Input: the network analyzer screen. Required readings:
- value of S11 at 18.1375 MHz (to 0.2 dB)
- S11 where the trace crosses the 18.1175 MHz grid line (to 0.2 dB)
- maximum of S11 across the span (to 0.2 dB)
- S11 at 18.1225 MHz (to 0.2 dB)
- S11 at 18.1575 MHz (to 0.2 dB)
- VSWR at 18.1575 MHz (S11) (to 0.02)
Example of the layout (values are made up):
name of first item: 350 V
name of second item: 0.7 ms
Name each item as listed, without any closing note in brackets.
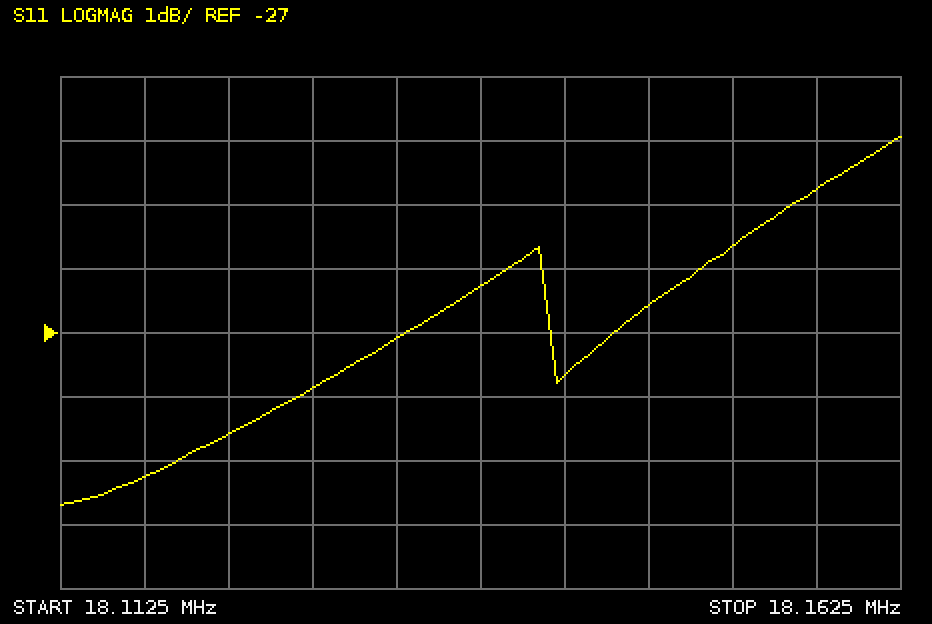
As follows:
value of S11 at 18.1375 MHz: -26.2 dB
S11 where the trace crosses the 18.1175 MHz grid line: -29.2 dB
maximum of S11 across the span: -24.0 dB
S11 at 18.1225 MHz: -28.6 dB
S11 at 18.1575 MHz: -24.8 dB
VSWR at 18.1575 MHz (S11): 1.12
